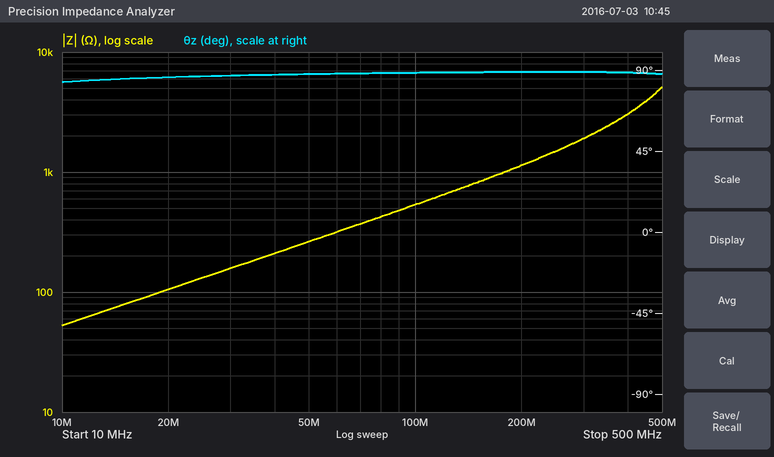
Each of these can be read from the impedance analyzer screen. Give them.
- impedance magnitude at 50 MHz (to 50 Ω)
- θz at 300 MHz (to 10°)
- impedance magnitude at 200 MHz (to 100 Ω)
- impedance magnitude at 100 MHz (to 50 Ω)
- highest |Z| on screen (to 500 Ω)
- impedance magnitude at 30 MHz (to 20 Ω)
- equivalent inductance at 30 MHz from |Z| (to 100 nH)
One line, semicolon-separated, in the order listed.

250 Ω; 90°; 1.1 kΩ; 550 Ω; 5.0 kΩ; 160 Ω; 800 nH
